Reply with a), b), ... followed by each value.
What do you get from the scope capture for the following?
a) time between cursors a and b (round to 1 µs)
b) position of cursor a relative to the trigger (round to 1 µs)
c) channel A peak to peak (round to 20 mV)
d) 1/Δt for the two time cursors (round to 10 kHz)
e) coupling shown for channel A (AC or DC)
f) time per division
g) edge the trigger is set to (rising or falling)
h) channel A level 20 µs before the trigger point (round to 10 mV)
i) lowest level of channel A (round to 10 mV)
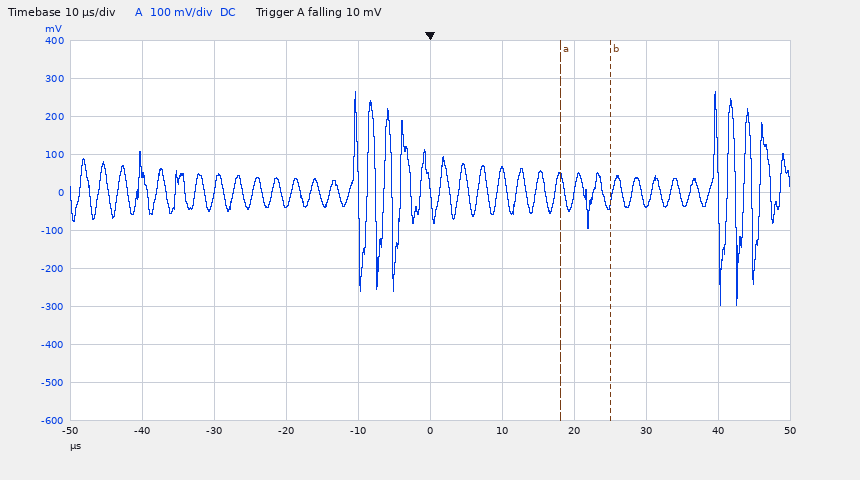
a) 7 µs
b) +18 µs
c) 560 mV
d) 140 kHz
e) DC
f) 10 µs
g) falling
h) -30 mV
i) -300 mV
